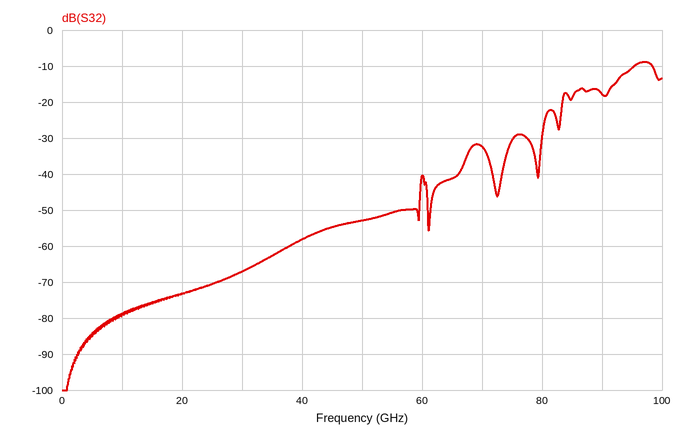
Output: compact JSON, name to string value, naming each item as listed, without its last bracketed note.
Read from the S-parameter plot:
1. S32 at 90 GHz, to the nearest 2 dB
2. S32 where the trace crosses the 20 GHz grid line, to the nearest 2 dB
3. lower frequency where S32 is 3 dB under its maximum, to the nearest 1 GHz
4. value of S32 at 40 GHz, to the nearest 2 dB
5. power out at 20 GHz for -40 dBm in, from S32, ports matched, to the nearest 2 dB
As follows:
{"S32 at 90 GHz, to the nearest 2 dB": "-18 dB", "S32 where the trace crosses the 20 GHz grid line, to the nearest 2 dB": "-74 dB", "lower frequency where S32 is 3 dB under its maximum, to the nearest 1 GHz": "94 GHz", "value of S32 at 40 GHz, to the nearest 2 dB": "-58 dB", "power out at 20 GHz for -40 dBm in, from S32, ports matched, to the nearest 2 dB": "-114 dBm"}
